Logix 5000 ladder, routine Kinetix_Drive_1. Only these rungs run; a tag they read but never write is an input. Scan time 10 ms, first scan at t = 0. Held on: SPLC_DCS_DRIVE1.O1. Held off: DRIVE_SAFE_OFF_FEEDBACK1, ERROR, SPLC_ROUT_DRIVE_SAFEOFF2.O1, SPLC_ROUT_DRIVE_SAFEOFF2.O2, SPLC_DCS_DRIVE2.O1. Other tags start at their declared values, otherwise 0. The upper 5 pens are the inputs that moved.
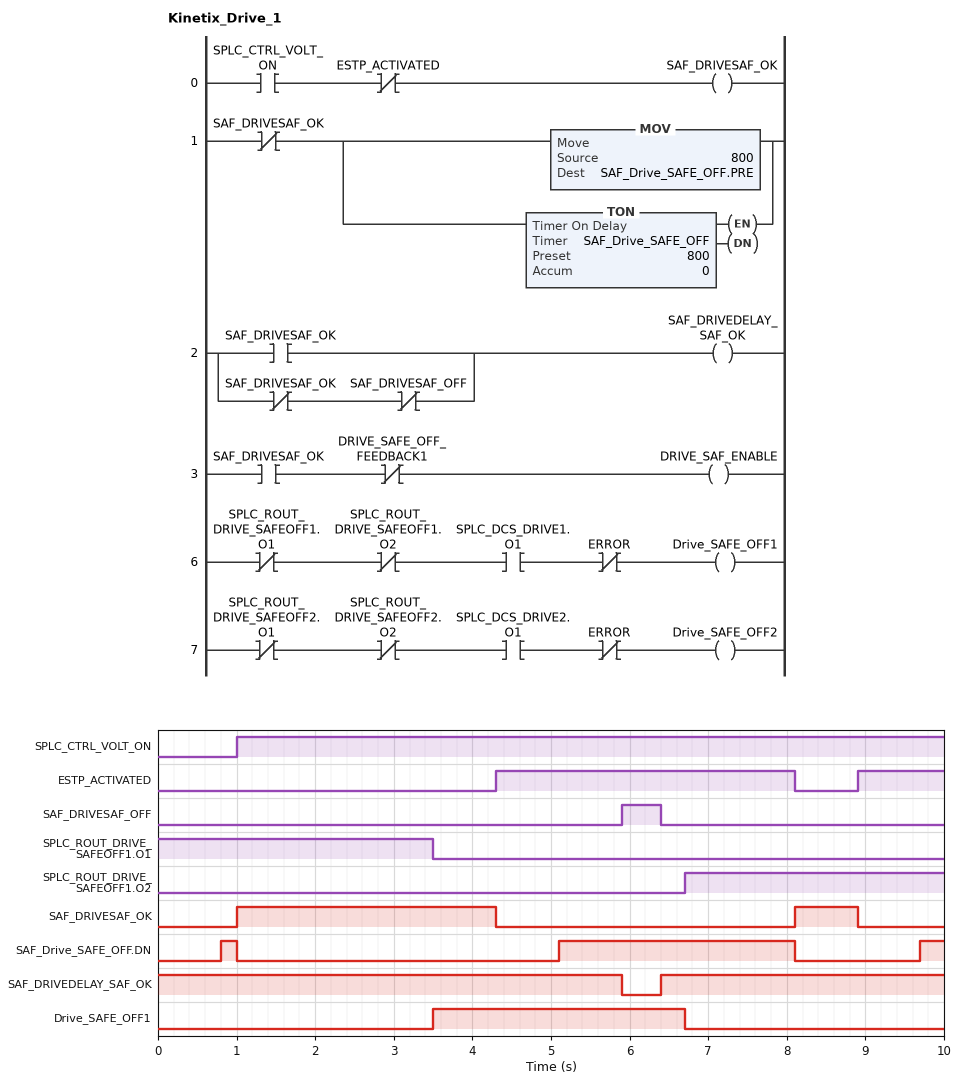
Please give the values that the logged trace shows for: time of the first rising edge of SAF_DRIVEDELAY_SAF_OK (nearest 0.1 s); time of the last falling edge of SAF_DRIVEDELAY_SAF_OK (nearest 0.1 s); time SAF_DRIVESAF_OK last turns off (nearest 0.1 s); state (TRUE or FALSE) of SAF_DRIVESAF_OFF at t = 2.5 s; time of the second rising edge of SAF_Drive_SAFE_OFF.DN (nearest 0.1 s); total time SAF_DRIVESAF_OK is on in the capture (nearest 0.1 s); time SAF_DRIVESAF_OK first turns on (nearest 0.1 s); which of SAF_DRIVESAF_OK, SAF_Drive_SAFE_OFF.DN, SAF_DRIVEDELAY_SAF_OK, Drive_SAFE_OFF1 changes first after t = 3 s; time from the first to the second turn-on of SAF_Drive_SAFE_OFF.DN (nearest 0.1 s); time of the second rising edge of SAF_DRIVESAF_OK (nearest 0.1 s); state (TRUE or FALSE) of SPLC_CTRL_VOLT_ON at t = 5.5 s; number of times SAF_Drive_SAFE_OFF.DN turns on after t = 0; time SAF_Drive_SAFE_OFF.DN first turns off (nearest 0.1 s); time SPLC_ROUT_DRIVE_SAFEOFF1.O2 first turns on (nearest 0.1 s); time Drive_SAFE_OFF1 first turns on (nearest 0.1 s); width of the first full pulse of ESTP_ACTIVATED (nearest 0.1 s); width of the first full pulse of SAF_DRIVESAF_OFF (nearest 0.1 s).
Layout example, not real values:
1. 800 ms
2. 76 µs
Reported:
1. 6.4 s
2. 5.9 s
3. 8.9 s
4. FALSE
5. 5.1 s
6. 4.1 s
7. 1.0 s
8. Drive_SAFE_OFF1
9. 4.3 s
10. 8.1 s
11. TRUE
12. 3
13. 1.0 s
14. 6.7 s
15. 3.5 s
16. 3.8 s
17. 0.5 s
